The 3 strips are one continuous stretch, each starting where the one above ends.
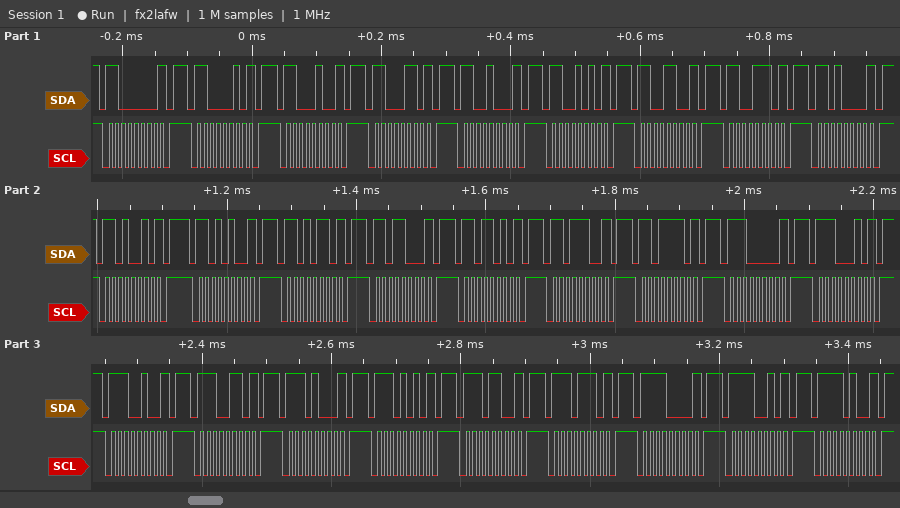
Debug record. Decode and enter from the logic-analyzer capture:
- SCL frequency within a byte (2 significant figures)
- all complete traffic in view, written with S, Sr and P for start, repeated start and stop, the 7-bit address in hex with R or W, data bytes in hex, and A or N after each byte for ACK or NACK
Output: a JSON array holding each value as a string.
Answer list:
["100 kHz", "S 60W N P S 61W N P S 62W N P S 63W N P S 64W N P S 65W N P S 66W N P S 67W N P S 68W N P S 69W N P S 6AW N P S 6BW N P S 6CW N P S 6DW N P S 6EW N P S 6FW N P S 70W N P S 71W N P S 72W N P S 73W N P S 74W N P S 75W N P S 76W N P S 77W N P S 78W N P S 79W N P S 7AW N P"]
